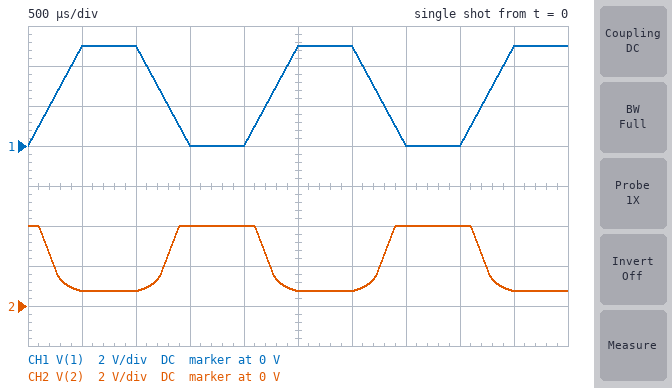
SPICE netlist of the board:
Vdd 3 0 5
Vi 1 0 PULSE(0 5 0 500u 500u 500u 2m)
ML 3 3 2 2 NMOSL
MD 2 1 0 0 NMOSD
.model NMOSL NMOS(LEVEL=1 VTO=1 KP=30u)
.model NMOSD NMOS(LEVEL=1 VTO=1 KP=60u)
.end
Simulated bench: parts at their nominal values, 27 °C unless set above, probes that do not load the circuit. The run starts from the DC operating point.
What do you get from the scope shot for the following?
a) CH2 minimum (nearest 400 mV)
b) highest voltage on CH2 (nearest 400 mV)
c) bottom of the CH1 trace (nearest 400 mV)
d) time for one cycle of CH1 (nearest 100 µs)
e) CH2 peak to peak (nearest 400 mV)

800 mV
4.0 V
0 V
2.0 ms
3.2 V
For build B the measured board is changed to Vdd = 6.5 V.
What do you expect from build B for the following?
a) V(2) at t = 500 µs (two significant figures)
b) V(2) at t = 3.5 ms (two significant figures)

1.3 V
5.5 V
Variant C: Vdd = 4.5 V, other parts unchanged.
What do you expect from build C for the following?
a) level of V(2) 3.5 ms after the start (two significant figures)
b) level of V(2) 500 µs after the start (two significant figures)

3.5 V
580 mV
